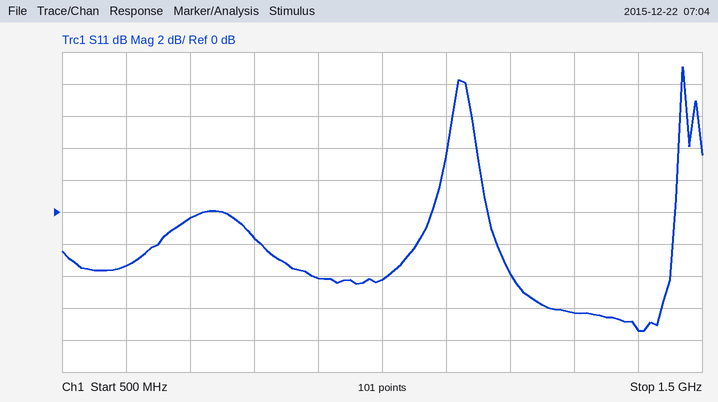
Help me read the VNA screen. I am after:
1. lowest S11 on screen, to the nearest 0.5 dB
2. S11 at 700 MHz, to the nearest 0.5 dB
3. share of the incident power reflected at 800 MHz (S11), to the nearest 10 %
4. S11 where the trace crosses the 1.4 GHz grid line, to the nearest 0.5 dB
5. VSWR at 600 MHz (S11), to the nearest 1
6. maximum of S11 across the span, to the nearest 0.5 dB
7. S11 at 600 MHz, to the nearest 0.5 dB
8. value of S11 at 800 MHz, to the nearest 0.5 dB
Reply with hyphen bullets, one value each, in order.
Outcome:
- -7.5 dB
- -0.5 dB
- 70 %
- -7.5 dB
- 5
- 9.0 dB
- -3.5 dB
- -1.5 dB
